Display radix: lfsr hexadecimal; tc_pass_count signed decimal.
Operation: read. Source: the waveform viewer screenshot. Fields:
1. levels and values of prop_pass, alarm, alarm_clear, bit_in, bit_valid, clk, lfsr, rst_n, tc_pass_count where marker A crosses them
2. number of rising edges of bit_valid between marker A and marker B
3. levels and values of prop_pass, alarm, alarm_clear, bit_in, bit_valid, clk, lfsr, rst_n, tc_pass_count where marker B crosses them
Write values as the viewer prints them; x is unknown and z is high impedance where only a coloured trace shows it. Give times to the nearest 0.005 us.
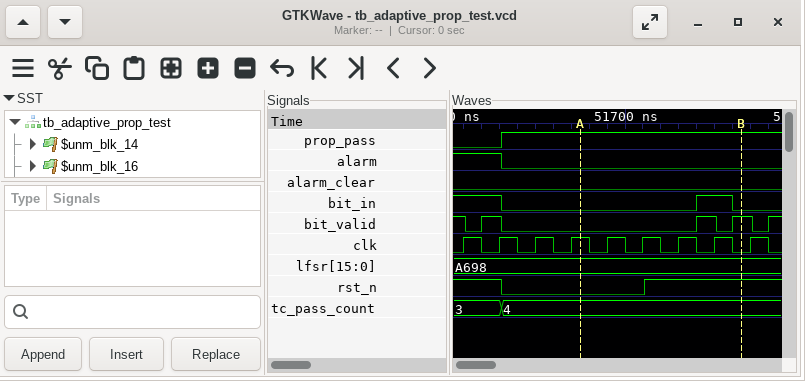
prop_pass=1, alarm=0, alarm_clear=0, bit_in=0, bit_valid=0, clk=1, lfsr=A698, rst_n=0, tc_pass_count=4
2
prop_pass=1, alarm=0, alarm_clear=0, bit_in=0, bit_valid=1, clk=0, lfsr=A698, rst_n=1, tc_pass_count=4
